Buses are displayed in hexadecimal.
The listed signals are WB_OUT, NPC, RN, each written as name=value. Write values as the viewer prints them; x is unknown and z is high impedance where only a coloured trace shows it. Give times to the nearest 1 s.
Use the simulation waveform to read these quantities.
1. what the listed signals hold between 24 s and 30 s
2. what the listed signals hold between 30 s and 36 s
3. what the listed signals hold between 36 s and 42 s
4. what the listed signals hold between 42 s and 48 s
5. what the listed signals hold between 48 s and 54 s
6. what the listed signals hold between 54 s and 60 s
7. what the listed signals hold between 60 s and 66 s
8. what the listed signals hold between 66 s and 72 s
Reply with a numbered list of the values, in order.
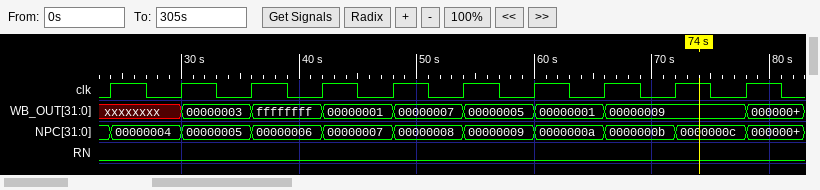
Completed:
1. WB_OUT=xxxxxxxx, NPC=00000004, RN=0
2. WB_OUT=00000003, NPC=00000005, RN=0
3. WB_OUT=ffffffff, NPC=00000006, RN=0
4. WB_OUT=00000001, NPC=00000007, RN=0
5. WB_OUT=00000007, NPC=00000008, RN=0
6. WB_OUT=00000005, NPC=00000009, RN=0
7. WB_OUT=00000001, NPC=0000000a, RN=0
8. WB_OUT=00000009, NPC=0000000b, RN=0
